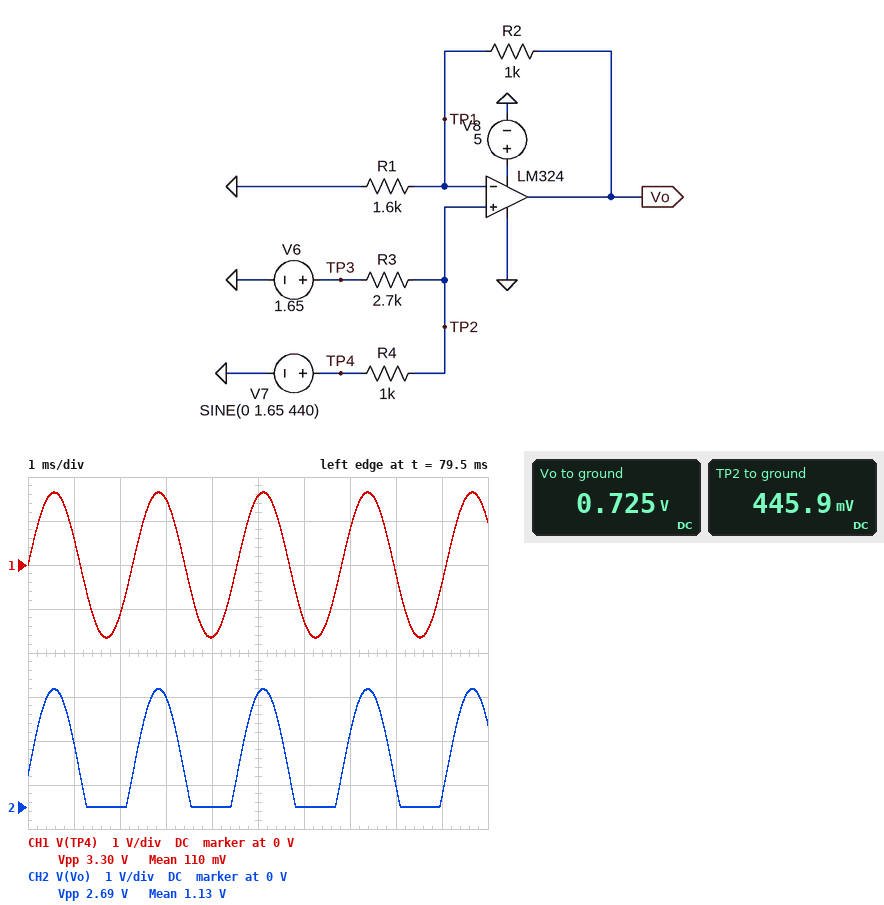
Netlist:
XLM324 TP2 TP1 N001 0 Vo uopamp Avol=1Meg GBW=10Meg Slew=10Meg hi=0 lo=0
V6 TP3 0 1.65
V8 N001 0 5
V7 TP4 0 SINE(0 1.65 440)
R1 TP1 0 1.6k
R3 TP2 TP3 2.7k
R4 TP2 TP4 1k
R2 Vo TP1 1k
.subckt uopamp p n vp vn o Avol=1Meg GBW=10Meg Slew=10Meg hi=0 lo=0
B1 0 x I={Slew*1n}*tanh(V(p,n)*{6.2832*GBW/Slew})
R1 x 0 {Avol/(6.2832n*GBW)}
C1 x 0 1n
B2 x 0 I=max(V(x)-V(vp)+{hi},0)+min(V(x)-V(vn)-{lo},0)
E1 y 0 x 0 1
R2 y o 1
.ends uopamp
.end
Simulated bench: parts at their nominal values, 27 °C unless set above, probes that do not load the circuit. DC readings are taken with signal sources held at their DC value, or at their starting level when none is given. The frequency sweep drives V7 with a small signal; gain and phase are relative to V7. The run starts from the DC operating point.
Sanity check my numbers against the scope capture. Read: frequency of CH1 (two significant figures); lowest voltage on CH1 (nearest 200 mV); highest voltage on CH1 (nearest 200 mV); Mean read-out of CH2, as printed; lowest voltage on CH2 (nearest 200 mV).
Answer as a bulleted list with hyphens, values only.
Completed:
- 440 Hz
- -1.6 V
- 1.6 V
- 1.13 V
- 0 V
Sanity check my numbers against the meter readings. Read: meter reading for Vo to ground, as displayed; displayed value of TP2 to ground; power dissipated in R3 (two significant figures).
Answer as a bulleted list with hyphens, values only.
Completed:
- 0.725 V
- 445.9 mV
- 540 µW
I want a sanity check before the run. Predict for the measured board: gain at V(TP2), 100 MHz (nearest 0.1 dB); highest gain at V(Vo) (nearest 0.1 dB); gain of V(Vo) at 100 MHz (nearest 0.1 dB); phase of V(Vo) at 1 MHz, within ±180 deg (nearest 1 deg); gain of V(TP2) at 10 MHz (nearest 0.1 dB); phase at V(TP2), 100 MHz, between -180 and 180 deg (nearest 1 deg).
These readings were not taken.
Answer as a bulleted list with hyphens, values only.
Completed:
- -2.7 dB
- 1.5 dB
- -22.8 dB
- -9 deg
- -2.7 dB
- 0 deg
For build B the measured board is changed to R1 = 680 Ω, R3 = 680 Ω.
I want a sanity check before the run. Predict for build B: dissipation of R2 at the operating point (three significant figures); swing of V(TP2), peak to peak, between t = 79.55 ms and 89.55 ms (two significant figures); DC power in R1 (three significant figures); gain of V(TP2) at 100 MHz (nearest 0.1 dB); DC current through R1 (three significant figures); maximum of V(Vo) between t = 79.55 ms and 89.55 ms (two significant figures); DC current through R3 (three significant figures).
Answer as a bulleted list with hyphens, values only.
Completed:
- 2.09 mW
- 1.3 V
- 1.42 mW
- -7.9 dB
- 1.44 mA
- 4.1 V
- 982 µA
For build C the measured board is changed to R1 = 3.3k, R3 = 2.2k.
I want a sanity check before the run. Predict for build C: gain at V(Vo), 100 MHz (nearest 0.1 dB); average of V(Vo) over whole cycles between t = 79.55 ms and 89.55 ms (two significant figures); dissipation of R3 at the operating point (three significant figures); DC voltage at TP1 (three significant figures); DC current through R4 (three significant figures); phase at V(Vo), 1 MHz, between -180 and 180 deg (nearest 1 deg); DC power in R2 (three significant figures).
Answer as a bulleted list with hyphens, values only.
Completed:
- -23.3 dB
- 850 mV
- 585 µW
- 516 mV
- 516 µA
- -7 deg
- 24.4 µW
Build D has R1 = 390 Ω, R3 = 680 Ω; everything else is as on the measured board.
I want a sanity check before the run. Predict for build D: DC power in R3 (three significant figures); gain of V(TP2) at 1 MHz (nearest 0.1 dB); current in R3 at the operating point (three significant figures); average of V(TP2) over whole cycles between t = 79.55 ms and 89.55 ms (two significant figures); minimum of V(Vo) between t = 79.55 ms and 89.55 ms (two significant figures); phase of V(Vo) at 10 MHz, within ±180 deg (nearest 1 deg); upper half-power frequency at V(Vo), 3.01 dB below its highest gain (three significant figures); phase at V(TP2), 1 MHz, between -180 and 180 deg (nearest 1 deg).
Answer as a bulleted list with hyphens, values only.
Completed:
- 656 µW
- -7.9 dB
- 982 µA
- 980 mV
- 1.1 V
- -74 deg
- 2.80 MHz
- 0 deg
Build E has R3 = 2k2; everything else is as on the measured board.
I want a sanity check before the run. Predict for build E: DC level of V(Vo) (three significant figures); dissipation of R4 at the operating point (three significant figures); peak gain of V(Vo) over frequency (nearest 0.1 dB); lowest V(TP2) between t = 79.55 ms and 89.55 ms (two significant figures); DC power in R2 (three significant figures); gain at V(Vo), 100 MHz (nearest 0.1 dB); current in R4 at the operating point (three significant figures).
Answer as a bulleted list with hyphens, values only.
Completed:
- 838 mV
- 266 µW
- 1.0 dB
- -620 mV
- 104 µW
- -23.3 dB
- 516 µA
